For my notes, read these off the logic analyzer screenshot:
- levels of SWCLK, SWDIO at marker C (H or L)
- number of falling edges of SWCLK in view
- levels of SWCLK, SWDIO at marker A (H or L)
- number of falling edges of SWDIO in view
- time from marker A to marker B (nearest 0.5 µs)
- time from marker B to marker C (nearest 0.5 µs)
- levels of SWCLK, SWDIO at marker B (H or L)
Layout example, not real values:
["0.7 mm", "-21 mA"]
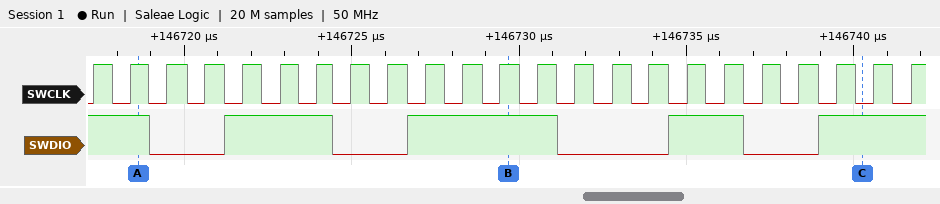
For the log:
["SWCLK=L, SWDIO=H", "22", "SWCLK=H, SWDIO=H", "4", "11 µs", "10.5 µs", "SWCLK=H, SWDIO=H"]
